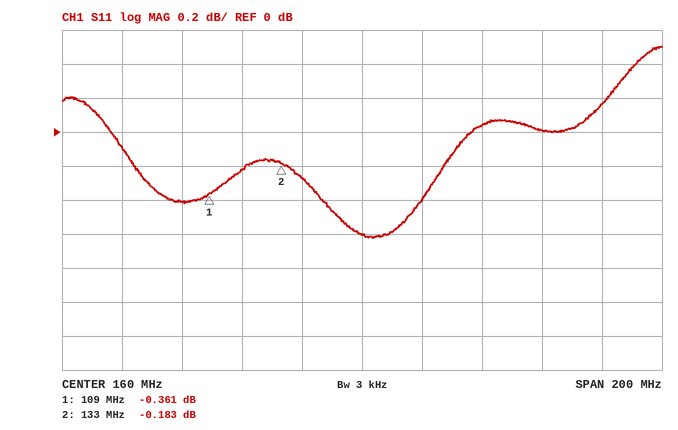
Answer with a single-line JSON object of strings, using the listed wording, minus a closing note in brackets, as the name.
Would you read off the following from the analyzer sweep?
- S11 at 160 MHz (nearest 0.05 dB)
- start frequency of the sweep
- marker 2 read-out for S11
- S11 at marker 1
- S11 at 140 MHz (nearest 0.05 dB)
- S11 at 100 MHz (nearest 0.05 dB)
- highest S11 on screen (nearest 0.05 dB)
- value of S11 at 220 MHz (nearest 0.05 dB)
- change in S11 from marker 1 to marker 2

{"S11 at 160 MHz": "-0.60 dB", "start frequency of the sweep": "60 MHz", "marker 2 read-out for S11": "-0.183 dB", "S11 at marker 1": "-0.361 dB", "S11 at 140 MHz": "-0.25 dB", "S11 at 100 MHz": "-0.40 dB", "highest S11 on screen": "0.50 dB", "value of S11 at 220 MHz": "0.00 dB", "change in S11 from marker 1 to marker 2": "0.178 dB"}
